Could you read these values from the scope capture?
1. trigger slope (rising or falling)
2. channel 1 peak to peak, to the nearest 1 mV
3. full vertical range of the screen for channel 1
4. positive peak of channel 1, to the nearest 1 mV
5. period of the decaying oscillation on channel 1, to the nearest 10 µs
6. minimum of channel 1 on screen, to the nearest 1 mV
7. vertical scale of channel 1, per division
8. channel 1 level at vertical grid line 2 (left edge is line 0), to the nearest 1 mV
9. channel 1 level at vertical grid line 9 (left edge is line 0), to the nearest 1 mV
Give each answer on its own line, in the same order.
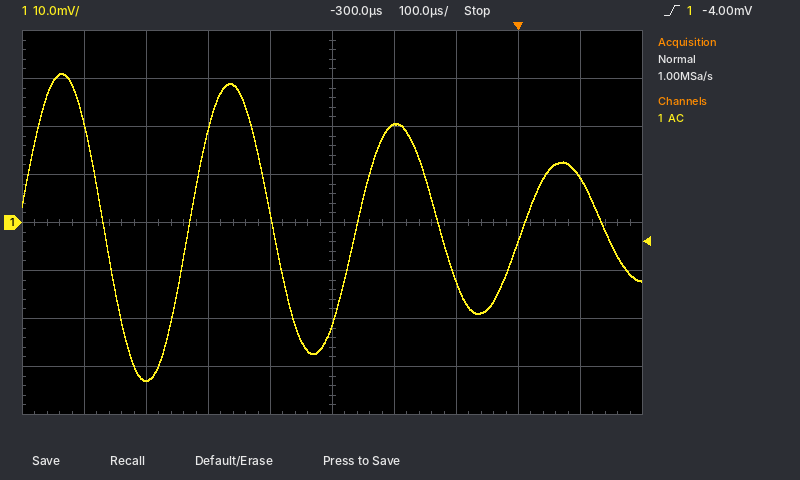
rising
64 mV
80 mV
31 mV
270 µs
-33 mV
10 mV
-33 mV
9 mV
